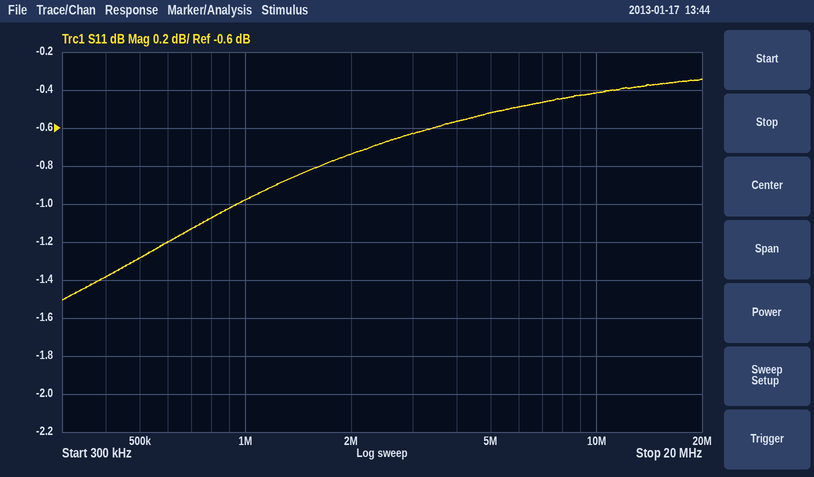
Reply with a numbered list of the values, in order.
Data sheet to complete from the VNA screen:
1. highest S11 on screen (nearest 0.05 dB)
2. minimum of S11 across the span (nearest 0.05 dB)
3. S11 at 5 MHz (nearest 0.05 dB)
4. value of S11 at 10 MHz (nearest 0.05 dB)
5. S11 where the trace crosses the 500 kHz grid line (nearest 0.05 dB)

1. -0.35 dB
2. -1.50 dB
3. -0.50 dB
4. -0.40 dB
5. -1.30 dB
